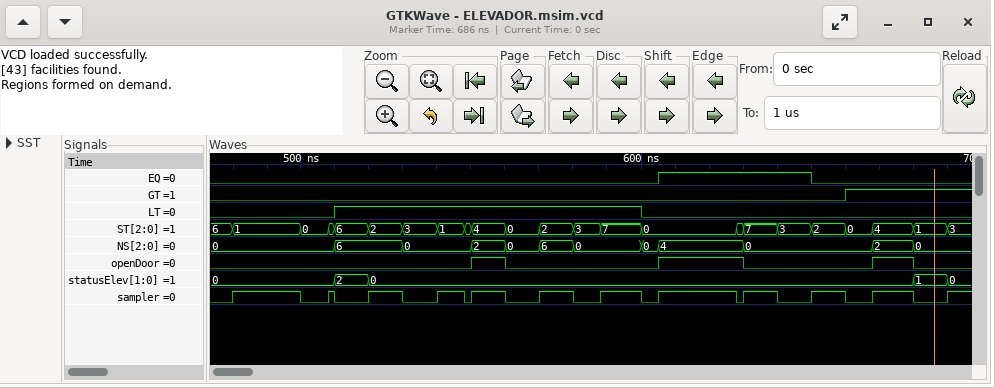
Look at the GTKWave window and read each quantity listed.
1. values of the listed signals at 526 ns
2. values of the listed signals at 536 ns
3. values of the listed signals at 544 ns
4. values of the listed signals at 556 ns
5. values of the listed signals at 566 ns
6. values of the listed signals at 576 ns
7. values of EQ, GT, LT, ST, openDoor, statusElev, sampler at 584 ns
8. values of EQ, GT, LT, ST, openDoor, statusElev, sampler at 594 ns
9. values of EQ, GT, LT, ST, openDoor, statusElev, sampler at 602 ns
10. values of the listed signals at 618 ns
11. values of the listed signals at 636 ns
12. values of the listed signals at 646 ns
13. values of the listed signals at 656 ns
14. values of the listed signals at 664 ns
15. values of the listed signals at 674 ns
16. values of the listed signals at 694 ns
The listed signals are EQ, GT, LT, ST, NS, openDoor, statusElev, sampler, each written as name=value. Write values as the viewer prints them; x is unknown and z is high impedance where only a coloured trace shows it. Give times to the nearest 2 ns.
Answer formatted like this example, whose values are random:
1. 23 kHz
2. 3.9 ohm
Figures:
1. EQ=0, GT=0, LT=1, ST=2, NS=6, openDoor=0, statusElev=0, sampler=1
2. EQ=0, GT=0, LT=1, ST=3, NS=0, openDoor=0, statusElev=0, sampler=0
3. EQ=0, GT=0, LT=1, ST=1, NS=0, openDoor=0, statusElev=0, sampler=1
4. EQ=0, GT=0, LT=1, ST=4, NS=2, openDoor=1, statusElev=0, sampler=1
5. EQ=0, GT=0, LT=1, ST=0, NS=0, openDoor=0, statusElev=0, sampler=0
6. EQ=0, GT=0, LT=1, ST=2, NS=6, openDoor=0, statusElev=0, sampler=1
7. EQ=0, GT=0, LT=1, ST=3, openDoor=0, statusElev=0, sampler=0
8. EQ=0, GT=0, LT=1, ST=7, openDoor=0, statusElev=0, sampler=1
9. EQ=0, GT=0, LT=0, ST=0, openDoor=0, statusElev=0, sampler=0
10. EQ=1, GT=0, LT=0, ST=0, NS=4, openDoor=1, statusElev=0, sampler=1
11. EQ=1, GT=0, LT=0, ST=7, NS=0, openDoor=0, statusElev=0, sampler=1
12. EQ=1, GT=0, LT=0, ST=3, NS=0, openDoor=0, statusElev=0, sampler=0
13. EQ=0, GT=0, LT=0, ST=2, NS=0, openDoor=0, statusElev=0, sampler=1
14. EQ=0, GT=1, LT=0, ST=0, NS=0, openDoor=0, statusElev=0, sampler=0
15. EQ=0, GT=1, LT=0, ST=4, NS=2, openDoor=1, statusElev=0, sampler=1
16. EQ=0, GT=1, LT=0, ST=3, NS=0, openDoor=0, statusElev=0, sampler=1
